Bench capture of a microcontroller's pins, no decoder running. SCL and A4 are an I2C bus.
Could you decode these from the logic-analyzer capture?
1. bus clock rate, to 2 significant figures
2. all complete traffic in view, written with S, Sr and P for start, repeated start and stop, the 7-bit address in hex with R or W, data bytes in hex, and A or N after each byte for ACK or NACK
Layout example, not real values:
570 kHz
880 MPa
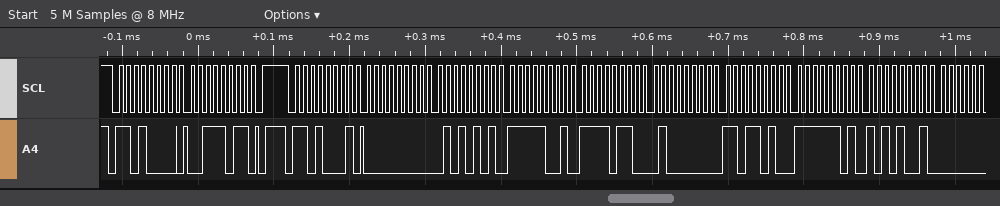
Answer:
100 kHz
S 68W A 3B A P S 68R A 00 A 55 A F9 A F6 A 40 A DA A FD A A9 A
